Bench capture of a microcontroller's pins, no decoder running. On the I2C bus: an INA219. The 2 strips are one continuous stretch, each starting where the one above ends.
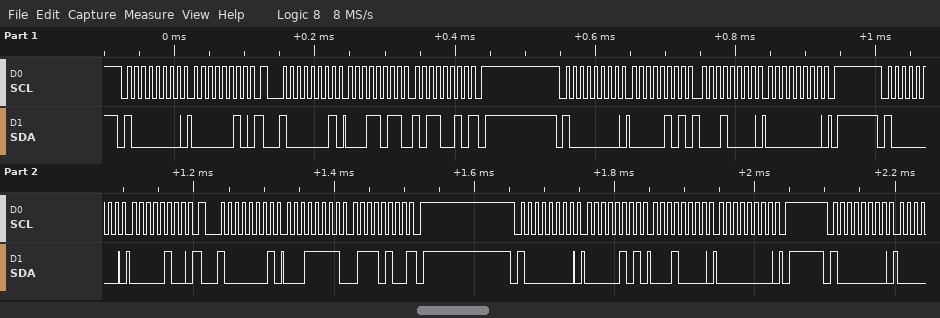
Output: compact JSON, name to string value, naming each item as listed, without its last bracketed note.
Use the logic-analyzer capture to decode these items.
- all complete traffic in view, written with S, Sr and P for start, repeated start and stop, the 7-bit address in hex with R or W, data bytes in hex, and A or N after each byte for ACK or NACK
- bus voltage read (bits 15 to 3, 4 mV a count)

{"all complete traffic in view, written with S, Sr and P for start, repeated start and stop, the 7-bit address in hex with R or W, data bytes in hex, and A or N after each byte for ACK or NACK": "S 40W A 02 A Sr 40R A 1B A B2 N P S 40W A 05 A 10 A 00 A P S 40W A 04 A Sr 40R A 1F A 74 N P S 40W A 05 A 10 A 00 A P S 40W A", "bus voltage read": "3.544 V"}
